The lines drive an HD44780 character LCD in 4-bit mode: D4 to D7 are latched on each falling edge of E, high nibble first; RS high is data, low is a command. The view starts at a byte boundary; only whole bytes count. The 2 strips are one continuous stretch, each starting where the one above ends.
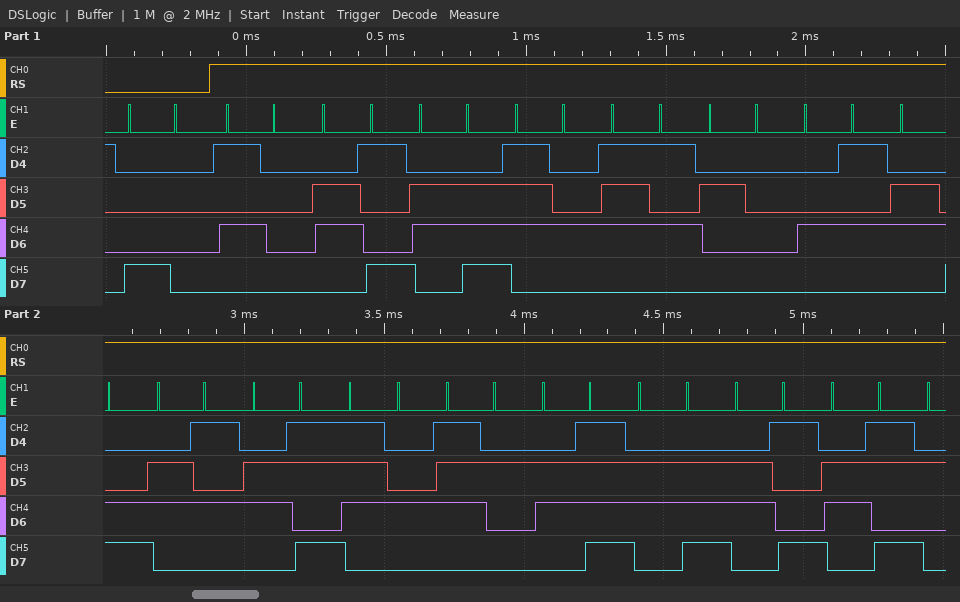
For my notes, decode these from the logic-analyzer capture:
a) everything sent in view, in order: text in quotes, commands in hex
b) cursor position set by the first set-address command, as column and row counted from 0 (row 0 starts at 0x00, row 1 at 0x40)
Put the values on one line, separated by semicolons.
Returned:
0x80 "Pintu Elektronik"; column 0, row 0
